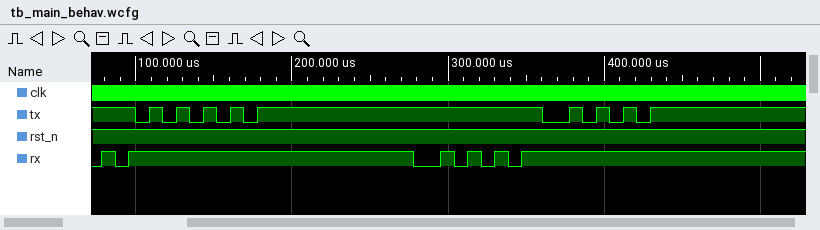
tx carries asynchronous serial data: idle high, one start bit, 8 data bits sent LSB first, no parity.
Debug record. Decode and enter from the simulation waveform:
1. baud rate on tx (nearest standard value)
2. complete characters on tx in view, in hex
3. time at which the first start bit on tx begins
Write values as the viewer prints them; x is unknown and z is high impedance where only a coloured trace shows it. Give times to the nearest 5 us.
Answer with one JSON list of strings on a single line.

["115200 baud", "55, AA", "100 us"]
